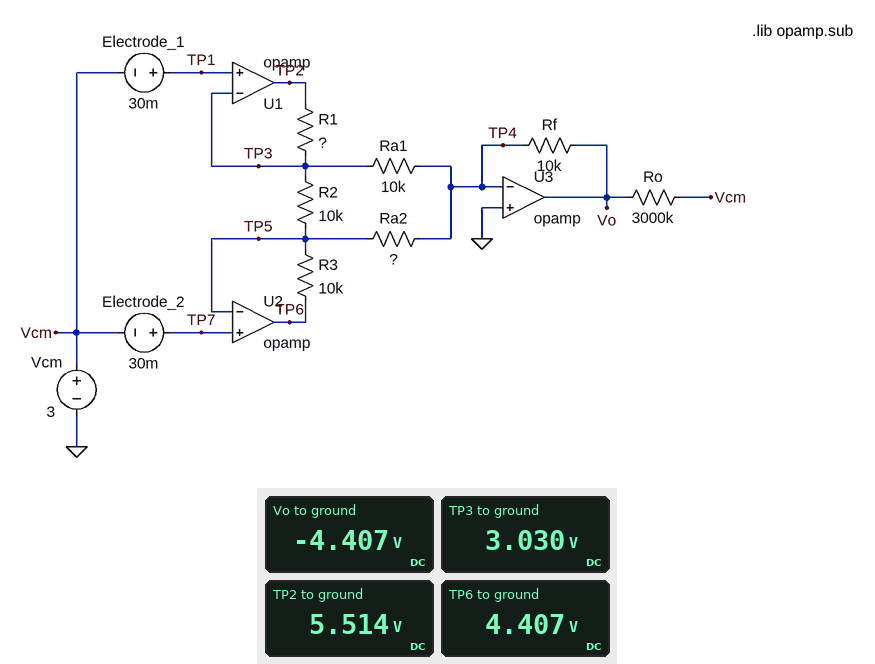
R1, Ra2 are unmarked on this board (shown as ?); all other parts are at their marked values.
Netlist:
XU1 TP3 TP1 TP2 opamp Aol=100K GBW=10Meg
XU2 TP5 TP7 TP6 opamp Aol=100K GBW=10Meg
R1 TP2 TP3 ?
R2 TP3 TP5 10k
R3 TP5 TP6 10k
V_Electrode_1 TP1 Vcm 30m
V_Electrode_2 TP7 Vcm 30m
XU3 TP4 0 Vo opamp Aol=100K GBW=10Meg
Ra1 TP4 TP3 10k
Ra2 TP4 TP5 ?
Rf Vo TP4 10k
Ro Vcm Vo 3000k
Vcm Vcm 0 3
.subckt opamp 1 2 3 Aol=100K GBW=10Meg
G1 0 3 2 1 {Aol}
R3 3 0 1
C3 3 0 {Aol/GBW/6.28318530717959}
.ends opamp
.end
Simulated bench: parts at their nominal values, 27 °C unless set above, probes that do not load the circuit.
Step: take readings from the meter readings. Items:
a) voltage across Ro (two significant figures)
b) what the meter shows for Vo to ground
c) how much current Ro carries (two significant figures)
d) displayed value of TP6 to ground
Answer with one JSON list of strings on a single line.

["7.4 V", "-4.407 V", "2.5 µA", "4.407 V"]
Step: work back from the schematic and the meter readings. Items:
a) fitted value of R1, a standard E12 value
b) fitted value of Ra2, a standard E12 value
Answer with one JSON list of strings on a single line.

["8.2 kΩ", "22 kΩ"]
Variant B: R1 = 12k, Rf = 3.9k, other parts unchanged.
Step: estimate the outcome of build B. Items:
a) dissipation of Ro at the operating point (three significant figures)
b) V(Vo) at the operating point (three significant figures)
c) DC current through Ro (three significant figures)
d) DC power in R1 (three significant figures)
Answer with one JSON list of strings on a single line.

["7.42 µW", "-1.72 V", "1.57 µA", "1.10 mW"]
